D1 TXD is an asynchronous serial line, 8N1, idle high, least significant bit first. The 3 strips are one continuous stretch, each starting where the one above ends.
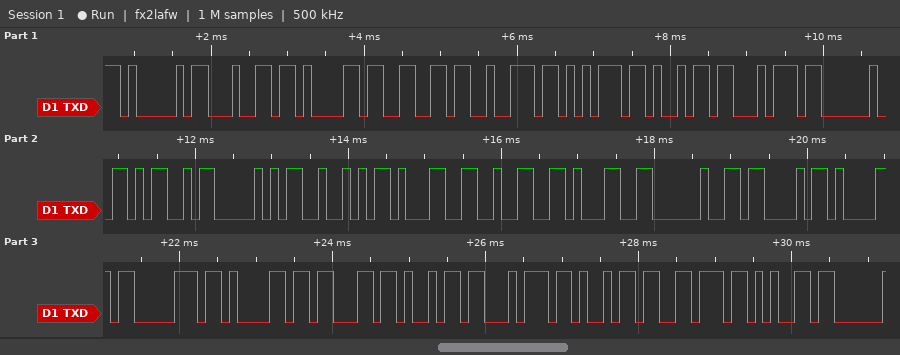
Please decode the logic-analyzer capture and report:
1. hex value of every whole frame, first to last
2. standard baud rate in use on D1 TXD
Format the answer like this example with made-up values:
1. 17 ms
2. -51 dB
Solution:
1. 0x41 0x64 0x61 0x66 0x72 0x75 0x69 0x74 0x20 0x4D 0x50 0x52 0x31 0x32 0x31 0x20 0x43 0x61 0x70 0x61 0x63 0x69 0x74 0x69 0x76 0x65
2. 9600 baud
